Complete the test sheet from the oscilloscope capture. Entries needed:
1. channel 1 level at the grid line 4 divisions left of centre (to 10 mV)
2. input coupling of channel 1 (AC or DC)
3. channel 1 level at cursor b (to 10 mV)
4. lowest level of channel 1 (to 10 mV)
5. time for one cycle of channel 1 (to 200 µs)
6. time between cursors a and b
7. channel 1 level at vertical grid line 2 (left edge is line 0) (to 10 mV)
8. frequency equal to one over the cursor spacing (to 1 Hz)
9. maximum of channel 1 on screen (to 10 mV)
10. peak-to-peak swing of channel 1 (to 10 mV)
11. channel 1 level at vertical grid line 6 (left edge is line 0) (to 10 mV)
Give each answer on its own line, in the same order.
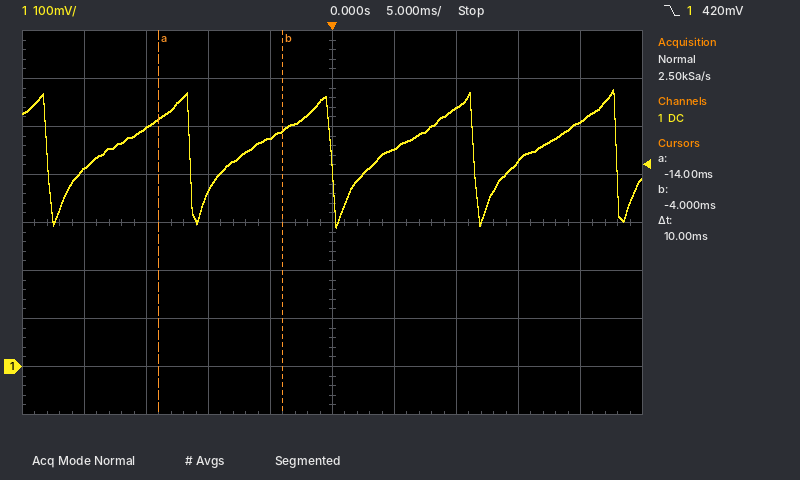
410 mV
DC
490 mV
290 mV
11.4 ms
10 ms
500 mV
100 Hz
580 mV
290 mV
450 mV
